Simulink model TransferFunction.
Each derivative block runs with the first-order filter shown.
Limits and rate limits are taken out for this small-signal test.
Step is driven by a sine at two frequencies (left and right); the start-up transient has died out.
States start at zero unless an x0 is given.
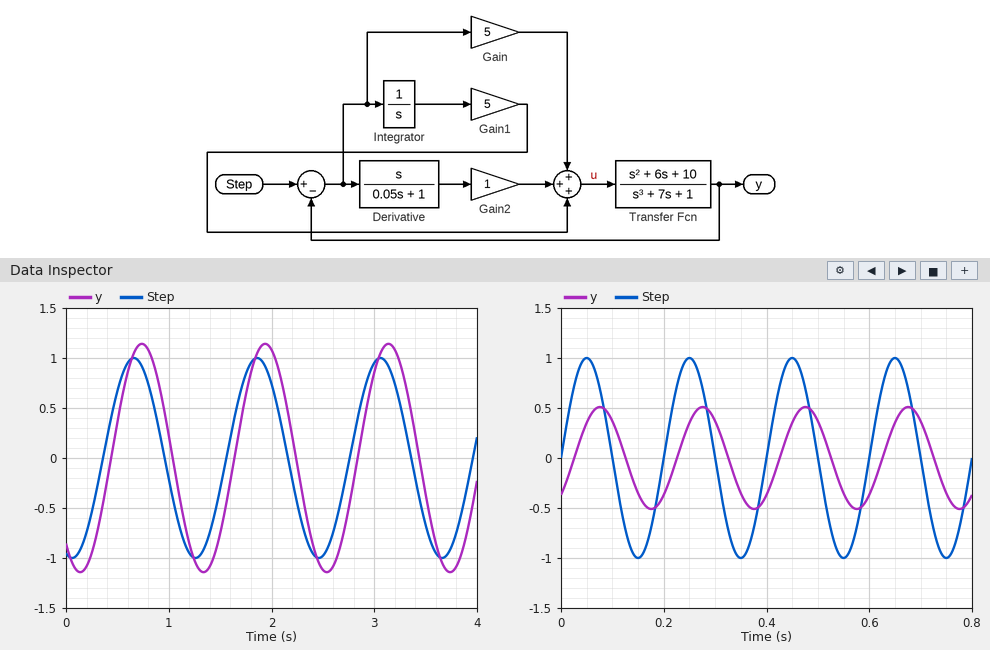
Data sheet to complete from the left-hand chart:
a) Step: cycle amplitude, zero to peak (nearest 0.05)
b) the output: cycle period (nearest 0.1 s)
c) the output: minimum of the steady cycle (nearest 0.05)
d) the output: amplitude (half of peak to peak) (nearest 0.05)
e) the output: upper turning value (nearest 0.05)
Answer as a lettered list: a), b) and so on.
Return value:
a) 1.00
b) 1.2 s
c) -1.15
d) 1.15
e) 1.15
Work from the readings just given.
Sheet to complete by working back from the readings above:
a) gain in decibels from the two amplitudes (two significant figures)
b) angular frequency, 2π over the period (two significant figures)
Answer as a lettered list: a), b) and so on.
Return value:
a) 1.2 dB
b) 5.2 rad/s
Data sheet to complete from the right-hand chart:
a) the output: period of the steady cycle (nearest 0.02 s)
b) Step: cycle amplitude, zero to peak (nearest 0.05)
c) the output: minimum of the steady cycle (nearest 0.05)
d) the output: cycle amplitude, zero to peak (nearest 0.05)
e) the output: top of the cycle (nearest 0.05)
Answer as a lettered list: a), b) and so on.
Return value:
a) 0.20 s
b) 1.00
c) -0.50
d) 0.50
e) 0.50
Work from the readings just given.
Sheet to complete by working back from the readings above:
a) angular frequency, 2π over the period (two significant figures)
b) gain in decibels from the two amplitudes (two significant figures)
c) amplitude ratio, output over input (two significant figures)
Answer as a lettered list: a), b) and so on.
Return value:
a) 31 rad/s
b) -6.0 dB
c) 0.50
